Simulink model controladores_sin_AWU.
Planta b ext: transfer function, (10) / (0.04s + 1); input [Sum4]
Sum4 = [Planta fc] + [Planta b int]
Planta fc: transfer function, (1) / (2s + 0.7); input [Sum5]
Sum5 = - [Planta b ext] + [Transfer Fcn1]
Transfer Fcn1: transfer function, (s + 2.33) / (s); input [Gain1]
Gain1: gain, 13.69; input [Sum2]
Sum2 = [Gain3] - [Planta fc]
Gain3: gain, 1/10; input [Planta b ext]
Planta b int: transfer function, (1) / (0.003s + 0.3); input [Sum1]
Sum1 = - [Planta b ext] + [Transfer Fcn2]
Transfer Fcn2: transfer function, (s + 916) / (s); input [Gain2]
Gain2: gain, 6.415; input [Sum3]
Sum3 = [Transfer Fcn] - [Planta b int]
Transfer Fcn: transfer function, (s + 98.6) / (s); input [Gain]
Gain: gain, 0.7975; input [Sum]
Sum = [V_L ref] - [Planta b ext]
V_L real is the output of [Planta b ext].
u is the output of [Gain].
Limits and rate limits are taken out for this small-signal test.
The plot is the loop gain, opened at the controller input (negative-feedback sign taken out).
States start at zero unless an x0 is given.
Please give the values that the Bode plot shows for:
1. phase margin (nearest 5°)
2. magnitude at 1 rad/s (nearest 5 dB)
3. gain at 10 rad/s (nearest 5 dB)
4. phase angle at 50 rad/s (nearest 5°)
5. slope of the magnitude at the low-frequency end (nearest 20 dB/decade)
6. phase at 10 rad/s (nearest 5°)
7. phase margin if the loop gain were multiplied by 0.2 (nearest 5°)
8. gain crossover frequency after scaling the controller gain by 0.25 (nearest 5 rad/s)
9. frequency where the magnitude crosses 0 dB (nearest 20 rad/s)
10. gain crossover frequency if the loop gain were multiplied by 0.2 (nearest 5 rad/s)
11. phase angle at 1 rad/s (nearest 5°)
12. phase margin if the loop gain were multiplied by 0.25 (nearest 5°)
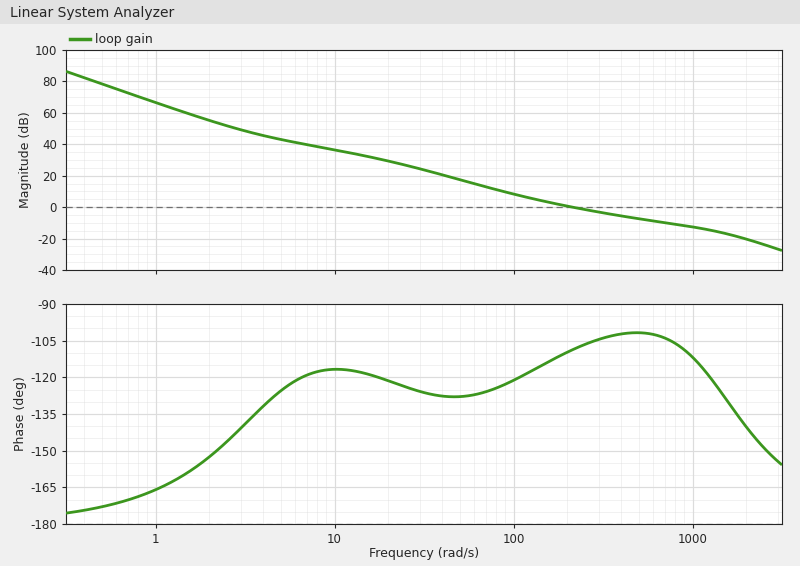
70°
65 dB
35 dB
-130°
-40 dB/decade
-115°
55°
75 rad/s
220 rad/s
65 rad/s
-165°
55°
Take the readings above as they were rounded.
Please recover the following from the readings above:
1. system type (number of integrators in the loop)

2
